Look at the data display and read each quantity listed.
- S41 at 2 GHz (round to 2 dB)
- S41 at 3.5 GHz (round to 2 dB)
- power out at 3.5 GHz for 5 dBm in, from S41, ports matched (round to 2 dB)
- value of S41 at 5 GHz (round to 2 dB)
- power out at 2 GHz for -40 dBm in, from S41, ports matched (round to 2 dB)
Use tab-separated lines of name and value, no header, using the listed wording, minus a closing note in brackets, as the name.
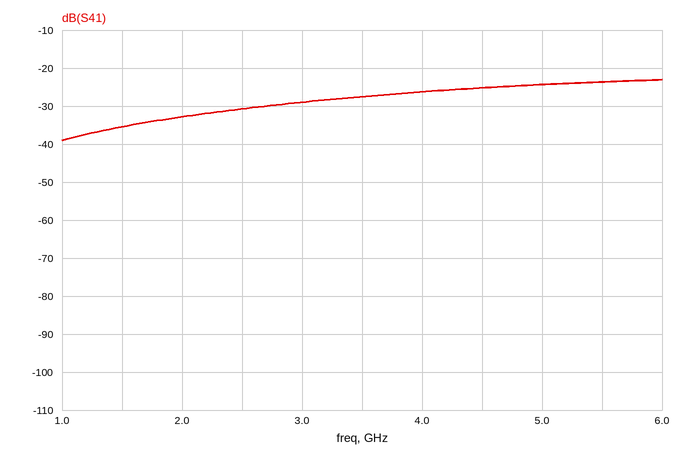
S41 at 2 GHz	-32 dB
S41 at 3.5 GHz	-28 dB
power out at 3.5 GHz for 5 dBm in, from S41, ports matched	-22 dBm
value of S41 at 5 GHz	-24 dB
power out at 2 GHz for -40 dBm in, from S41, ports matched	-72 dBm
